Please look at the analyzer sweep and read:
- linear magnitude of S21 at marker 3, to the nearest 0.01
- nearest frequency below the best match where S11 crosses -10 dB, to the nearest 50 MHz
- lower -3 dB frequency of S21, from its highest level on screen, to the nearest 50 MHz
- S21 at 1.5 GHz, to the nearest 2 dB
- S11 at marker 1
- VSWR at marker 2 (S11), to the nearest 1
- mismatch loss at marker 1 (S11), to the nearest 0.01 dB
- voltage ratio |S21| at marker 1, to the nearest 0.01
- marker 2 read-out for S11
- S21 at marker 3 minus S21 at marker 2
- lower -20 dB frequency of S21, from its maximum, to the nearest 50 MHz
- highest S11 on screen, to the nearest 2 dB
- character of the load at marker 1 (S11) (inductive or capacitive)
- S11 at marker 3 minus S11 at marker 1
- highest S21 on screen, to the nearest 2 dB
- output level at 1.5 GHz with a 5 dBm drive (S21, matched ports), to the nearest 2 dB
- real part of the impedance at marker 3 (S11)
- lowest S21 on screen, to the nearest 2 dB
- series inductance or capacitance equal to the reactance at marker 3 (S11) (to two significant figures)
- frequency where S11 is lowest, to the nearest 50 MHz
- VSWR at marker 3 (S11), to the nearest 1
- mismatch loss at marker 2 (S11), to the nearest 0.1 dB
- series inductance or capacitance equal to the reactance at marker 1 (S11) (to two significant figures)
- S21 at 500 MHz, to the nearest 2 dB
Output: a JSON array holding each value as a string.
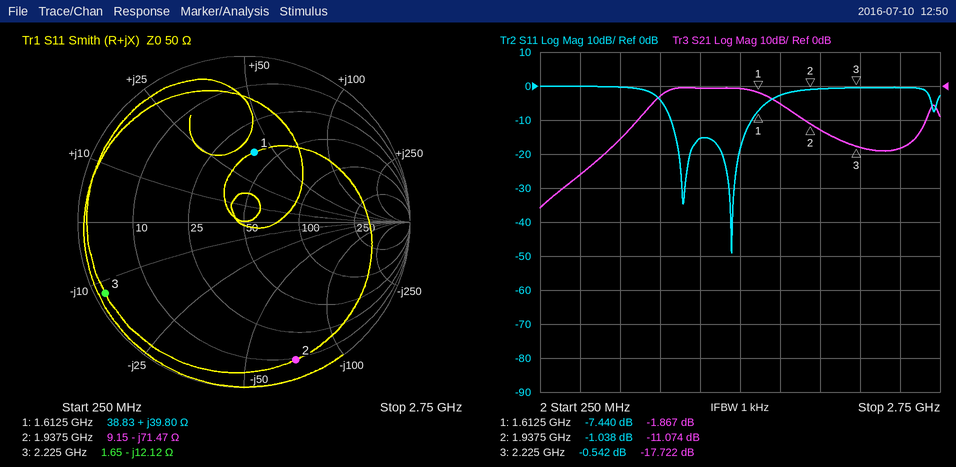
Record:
["0.13", "1.05 GHz", "1.00 GHz", "0 dB", "-7.440 dB", "17", "0.86 dB", "0.81", "-1.038 dB", "-6.648 dB", "650 MHz", "0 dB", "inductive", "6.898 dB", "0 dB", "4 dBm", "1.65 Ω", "-36 dB", "5.9 pF", "1.45 GHz", "32", "6.7 dB", "3.9 nH", "-26 dB"]
